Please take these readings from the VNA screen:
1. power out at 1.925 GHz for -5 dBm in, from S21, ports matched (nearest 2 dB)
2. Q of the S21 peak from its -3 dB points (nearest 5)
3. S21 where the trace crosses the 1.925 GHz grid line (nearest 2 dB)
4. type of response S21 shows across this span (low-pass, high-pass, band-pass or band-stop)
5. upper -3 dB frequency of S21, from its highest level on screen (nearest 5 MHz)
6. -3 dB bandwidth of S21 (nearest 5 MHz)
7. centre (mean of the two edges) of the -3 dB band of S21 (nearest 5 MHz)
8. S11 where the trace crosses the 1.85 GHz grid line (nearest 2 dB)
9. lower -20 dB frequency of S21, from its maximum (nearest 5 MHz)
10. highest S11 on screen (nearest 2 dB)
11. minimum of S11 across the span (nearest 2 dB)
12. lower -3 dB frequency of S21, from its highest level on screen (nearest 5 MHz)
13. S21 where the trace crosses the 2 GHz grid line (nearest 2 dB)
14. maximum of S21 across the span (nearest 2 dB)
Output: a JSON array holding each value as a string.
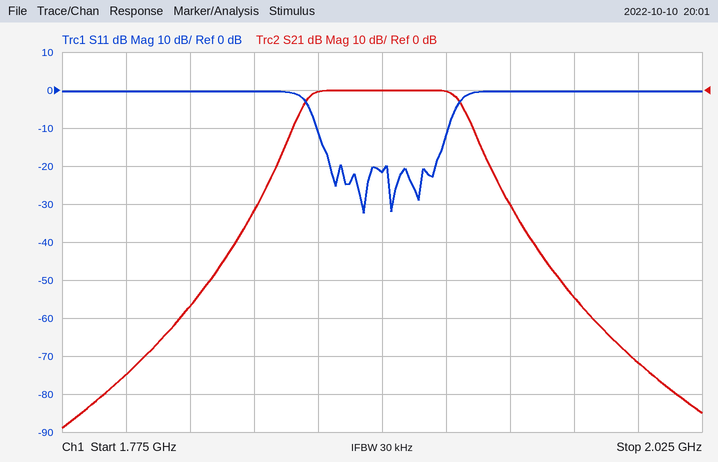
["-6 dBm", "30", "0 dB", "band-pass", "1.930 GHz", "60 MHz", "1.900 GHz", "0 dB", "1.860 GHz", "0 dB", "-32 dB", "1.870 GHz", "-72 dB", "0 dB"]
